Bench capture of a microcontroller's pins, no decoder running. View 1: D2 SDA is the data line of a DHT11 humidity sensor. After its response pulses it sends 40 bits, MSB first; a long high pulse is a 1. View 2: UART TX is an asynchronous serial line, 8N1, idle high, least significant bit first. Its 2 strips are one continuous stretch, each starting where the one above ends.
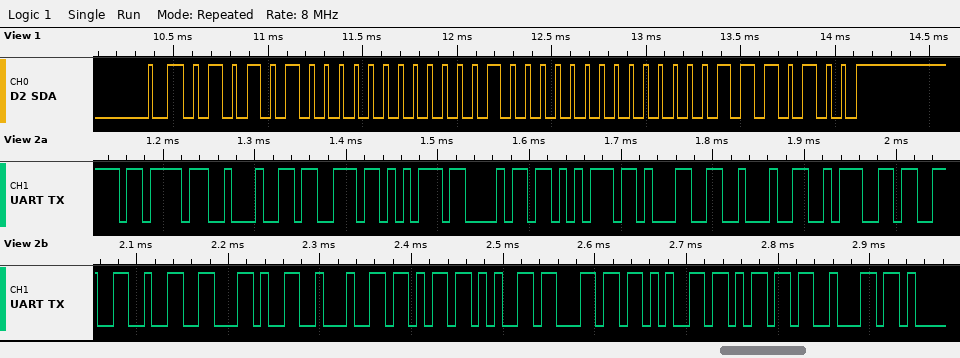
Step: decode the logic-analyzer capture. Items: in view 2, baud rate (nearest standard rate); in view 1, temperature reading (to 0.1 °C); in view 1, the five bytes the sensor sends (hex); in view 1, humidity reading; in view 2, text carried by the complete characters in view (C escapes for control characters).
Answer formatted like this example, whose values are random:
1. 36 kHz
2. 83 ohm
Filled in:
1. 115200 baud
2. 32.0 °C
3. 54 00 20 00 74
4. 84 %
5. "{\"suhu1\":32,\"kelemb"
